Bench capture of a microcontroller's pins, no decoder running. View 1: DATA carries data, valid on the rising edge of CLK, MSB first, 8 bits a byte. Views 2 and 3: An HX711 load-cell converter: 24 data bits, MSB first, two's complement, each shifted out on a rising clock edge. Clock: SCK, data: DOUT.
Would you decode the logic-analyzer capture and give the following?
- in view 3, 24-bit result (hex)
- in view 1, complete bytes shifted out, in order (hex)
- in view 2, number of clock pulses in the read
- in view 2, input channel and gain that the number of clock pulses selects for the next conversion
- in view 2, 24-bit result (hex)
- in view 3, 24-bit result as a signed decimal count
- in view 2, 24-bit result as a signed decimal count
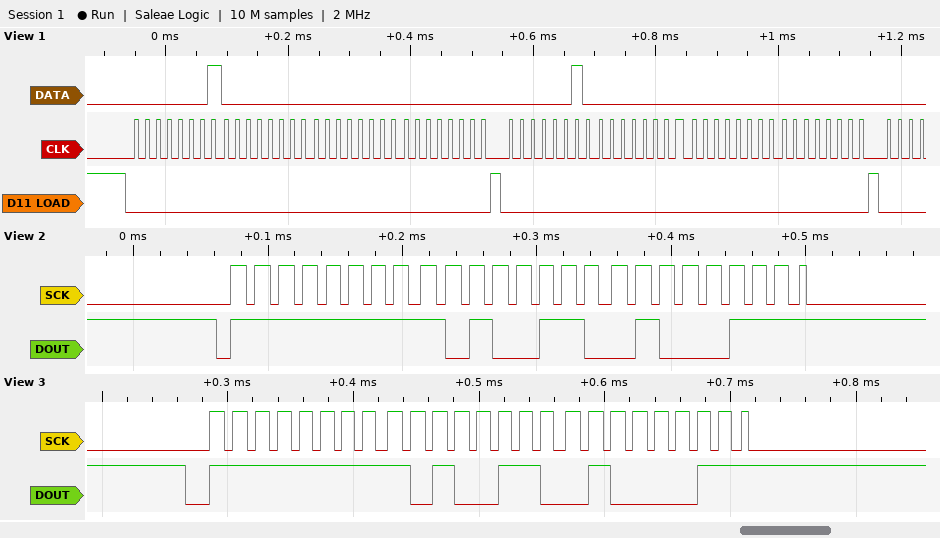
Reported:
0xFFA643
01 00 00 00 02 00 00 00
25
channel A, gain 128
0xFFA647
-22973
-22969
